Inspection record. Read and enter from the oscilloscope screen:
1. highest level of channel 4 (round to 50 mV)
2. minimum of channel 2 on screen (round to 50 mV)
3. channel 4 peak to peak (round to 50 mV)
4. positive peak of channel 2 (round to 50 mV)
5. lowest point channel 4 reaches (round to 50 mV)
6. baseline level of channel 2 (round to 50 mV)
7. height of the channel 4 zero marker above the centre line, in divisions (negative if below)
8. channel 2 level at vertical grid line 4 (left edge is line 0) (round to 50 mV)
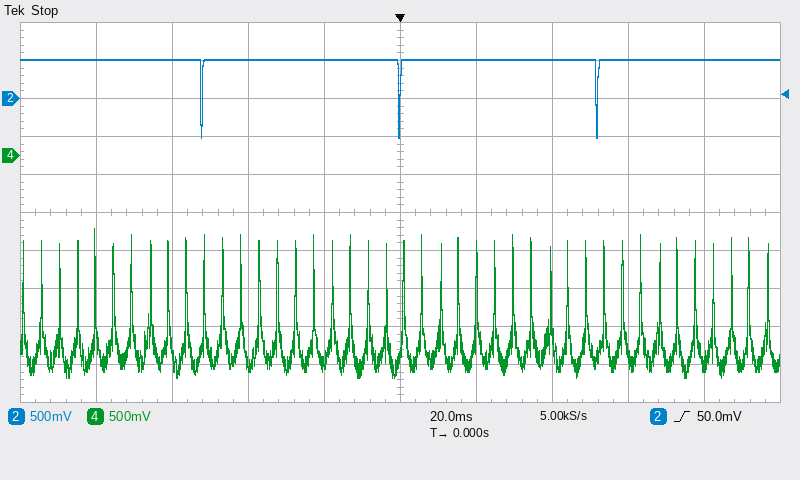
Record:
-950 mV
-500 mV
1.95 V
500 mV
-2.90 V
500 mV
+1.5 div
500 mV
